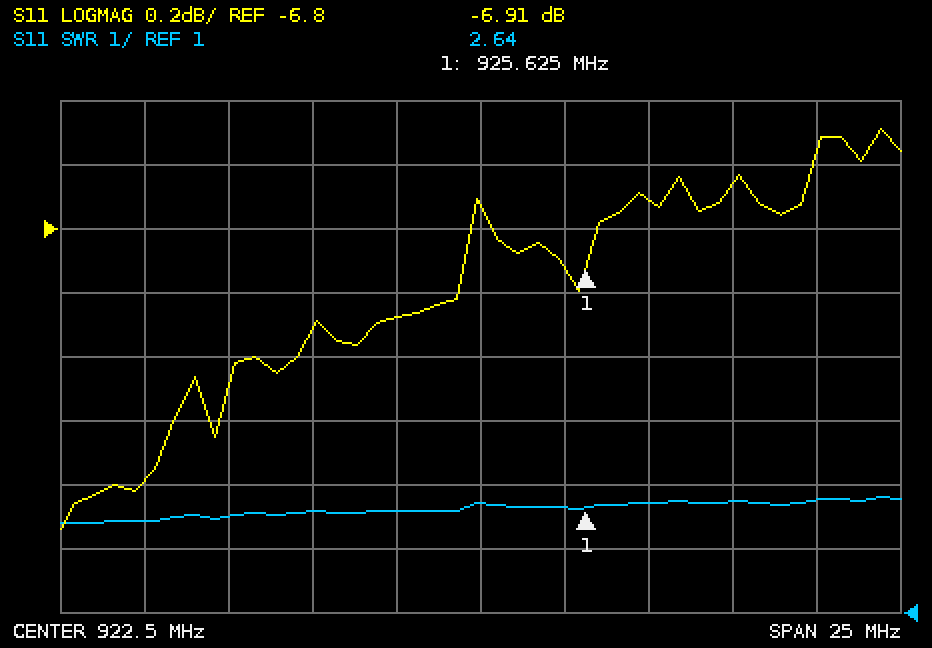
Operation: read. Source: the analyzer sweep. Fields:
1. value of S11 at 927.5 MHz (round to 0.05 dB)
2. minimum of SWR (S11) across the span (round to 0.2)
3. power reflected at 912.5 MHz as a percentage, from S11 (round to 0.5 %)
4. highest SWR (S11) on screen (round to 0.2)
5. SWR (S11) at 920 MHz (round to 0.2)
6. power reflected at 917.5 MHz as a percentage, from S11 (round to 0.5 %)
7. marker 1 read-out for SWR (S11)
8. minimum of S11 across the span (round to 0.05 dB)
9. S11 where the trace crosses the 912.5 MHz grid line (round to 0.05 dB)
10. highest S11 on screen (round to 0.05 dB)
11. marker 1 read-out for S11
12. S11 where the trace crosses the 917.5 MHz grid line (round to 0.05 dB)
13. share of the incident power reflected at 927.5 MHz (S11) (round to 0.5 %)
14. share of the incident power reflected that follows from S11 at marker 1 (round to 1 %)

-6.70 dB
2.4
17.5 %
2.8
2.6
19.5 %
2.64
-7.75 dB
-7.60 dB
-6.50 dB
-6.91 dB
-7.10 dB
21.5 %
20 %
